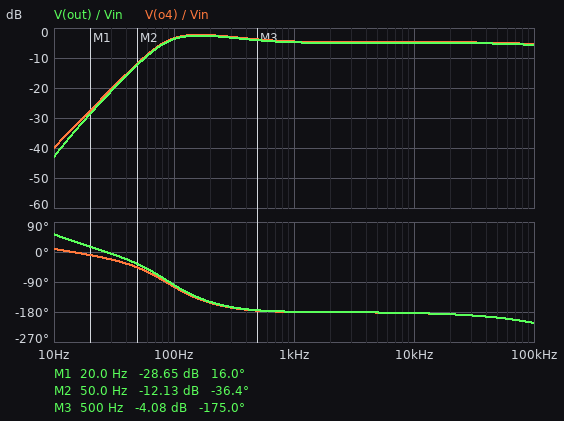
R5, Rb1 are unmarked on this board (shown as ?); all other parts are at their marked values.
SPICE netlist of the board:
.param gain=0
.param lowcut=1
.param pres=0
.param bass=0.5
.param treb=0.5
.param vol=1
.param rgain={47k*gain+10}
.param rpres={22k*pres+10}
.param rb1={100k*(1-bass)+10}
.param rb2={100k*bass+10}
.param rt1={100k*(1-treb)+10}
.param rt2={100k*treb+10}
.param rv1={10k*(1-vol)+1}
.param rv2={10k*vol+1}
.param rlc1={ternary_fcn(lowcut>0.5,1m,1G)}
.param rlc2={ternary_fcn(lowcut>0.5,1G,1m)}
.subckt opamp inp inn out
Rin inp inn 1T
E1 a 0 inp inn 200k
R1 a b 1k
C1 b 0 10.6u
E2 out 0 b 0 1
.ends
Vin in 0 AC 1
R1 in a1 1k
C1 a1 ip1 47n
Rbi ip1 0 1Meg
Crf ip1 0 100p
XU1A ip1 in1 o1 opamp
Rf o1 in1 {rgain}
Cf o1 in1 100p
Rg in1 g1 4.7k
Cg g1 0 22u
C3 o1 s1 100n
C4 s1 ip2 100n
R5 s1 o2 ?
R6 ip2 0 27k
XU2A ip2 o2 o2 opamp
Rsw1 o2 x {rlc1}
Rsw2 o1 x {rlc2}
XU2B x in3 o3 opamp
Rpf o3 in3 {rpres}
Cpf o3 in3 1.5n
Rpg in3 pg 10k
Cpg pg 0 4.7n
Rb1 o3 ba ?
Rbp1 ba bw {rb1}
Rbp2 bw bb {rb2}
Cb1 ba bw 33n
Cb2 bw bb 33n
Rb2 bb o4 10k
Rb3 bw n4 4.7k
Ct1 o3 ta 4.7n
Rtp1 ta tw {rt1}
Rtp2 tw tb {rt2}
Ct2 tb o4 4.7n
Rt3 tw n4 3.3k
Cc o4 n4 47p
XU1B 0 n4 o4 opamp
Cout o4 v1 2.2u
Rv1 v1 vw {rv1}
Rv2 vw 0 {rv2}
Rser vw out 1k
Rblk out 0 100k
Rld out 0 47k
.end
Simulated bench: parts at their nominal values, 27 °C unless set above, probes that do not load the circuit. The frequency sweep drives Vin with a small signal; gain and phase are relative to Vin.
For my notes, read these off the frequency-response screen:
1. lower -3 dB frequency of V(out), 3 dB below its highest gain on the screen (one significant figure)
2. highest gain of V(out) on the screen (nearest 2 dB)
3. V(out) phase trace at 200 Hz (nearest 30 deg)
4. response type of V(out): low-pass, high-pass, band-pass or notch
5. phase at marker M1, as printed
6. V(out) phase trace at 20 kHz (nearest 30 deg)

80 Hz
-2 dB
-150 deg
high-pass
16.0 deg
-180 deg
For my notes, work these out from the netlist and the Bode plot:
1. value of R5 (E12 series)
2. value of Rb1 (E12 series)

12 kΩ
22 kΩ
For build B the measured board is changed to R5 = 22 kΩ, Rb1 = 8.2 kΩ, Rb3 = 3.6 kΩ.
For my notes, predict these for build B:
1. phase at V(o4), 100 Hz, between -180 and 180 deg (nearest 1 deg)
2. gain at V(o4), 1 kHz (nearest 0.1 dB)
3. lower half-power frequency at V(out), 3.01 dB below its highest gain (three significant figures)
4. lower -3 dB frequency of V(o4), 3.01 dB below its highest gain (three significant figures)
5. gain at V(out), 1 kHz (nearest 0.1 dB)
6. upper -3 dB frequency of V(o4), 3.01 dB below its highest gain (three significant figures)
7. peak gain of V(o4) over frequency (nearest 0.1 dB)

-113 deg
1.0 dB
110 Hz
109 Hz
0.8 dB
217 kHz
1.3 dB
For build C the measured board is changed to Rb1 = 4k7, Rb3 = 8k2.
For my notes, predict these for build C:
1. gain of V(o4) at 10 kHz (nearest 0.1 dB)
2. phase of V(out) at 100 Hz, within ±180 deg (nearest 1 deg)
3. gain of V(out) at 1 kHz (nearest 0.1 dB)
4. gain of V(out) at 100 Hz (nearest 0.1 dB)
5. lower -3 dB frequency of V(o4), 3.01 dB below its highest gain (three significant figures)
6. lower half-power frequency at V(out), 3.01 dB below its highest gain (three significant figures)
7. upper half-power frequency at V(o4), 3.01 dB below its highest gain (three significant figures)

4.5 dB
-90 deg
3.1 dB
-1.0 dB
308 Hz
309 Hz
141 kHz
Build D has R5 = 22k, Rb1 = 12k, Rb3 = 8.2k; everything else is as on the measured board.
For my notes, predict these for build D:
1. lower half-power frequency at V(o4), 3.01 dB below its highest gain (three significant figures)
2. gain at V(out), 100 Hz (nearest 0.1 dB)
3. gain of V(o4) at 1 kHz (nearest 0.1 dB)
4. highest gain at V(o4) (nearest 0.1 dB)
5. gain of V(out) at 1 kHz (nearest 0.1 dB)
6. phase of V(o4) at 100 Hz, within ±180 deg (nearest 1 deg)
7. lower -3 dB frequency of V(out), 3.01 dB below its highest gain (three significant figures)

81.1 Hz
-3.0 dB
-1.0 dB
-0.8 dB
-1.3 dB
-115 deg
81.8 Hz
